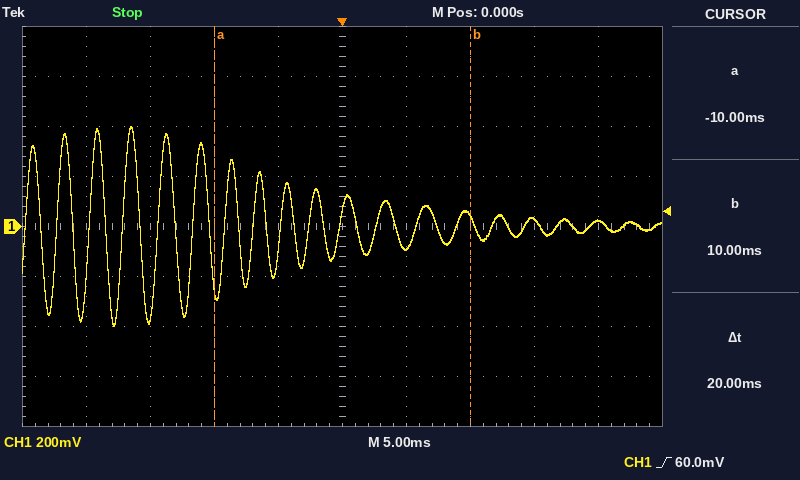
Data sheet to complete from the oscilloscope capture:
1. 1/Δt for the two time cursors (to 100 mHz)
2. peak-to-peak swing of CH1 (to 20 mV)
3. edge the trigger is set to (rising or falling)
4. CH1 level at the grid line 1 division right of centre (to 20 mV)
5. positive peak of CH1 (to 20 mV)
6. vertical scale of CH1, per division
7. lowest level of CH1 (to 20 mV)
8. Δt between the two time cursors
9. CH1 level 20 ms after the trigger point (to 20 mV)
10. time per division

50.0 Hz
800 mV
rising
-80 mV
400 mV
200 mV
-400 mV
20 ms
20 mV
5 ms
